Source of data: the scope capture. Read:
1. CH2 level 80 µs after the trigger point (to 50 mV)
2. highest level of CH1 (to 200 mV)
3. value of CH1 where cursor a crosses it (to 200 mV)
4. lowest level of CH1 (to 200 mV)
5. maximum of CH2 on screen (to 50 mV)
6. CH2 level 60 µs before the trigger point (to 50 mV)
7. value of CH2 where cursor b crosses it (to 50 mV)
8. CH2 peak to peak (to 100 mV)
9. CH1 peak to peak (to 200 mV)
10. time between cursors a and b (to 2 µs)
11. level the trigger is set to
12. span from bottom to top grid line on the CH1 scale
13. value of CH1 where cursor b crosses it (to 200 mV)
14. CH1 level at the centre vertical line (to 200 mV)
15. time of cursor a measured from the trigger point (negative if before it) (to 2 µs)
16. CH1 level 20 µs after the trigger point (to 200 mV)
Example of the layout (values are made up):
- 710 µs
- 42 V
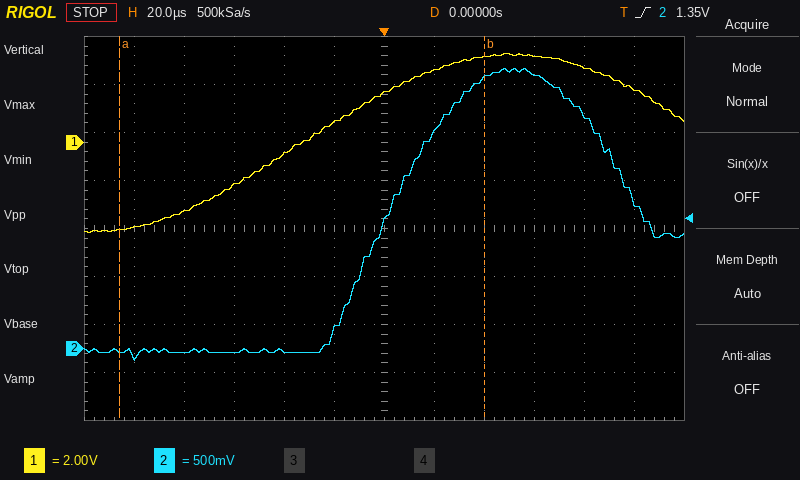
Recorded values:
- 2.45 V
- 3.6 V
- -3.6 V
- -3.8 V
- 2.90 V
- -50 mV
- 2.80 V
- 3.00 V
- 7.4 V
- 146 µs
- 1.35 V
- 16 V
- 3.6 V
- 2.0 V
- -106 µs
- 3.0 V
